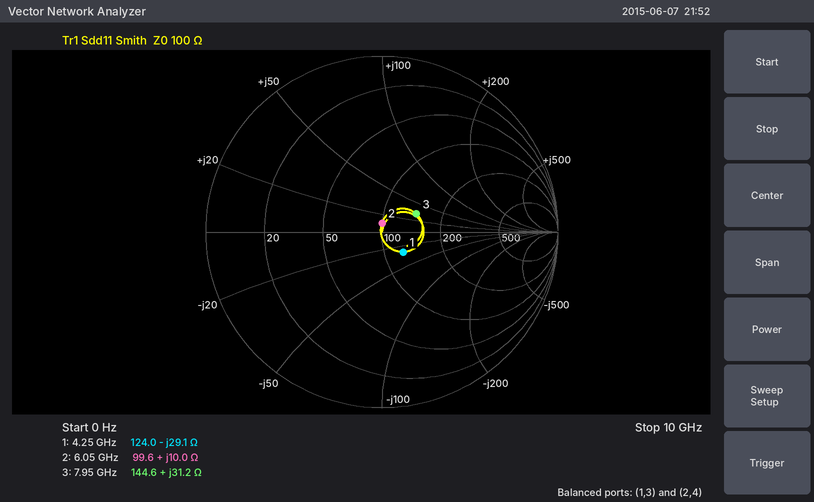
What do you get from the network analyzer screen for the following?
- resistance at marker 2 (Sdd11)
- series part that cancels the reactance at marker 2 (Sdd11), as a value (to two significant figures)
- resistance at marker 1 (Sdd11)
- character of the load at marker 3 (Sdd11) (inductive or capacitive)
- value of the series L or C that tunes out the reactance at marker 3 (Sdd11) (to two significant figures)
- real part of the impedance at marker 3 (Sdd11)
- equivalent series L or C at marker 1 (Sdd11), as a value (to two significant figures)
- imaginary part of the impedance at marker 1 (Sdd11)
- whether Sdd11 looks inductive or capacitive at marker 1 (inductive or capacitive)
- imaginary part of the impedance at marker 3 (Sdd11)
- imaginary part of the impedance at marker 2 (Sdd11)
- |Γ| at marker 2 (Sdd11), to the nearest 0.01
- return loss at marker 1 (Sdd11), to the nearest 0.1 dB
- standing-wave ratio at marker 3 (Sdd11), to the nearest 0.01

99.6 Ω
2.6 pF
124.0 Ω
inductive
640 fF
144.6 Ω
1.3 pF
-29.1 Ω
capacitive
+31.2 Ω
+10.0 Ω
0.05
15.5 dB
1.57
